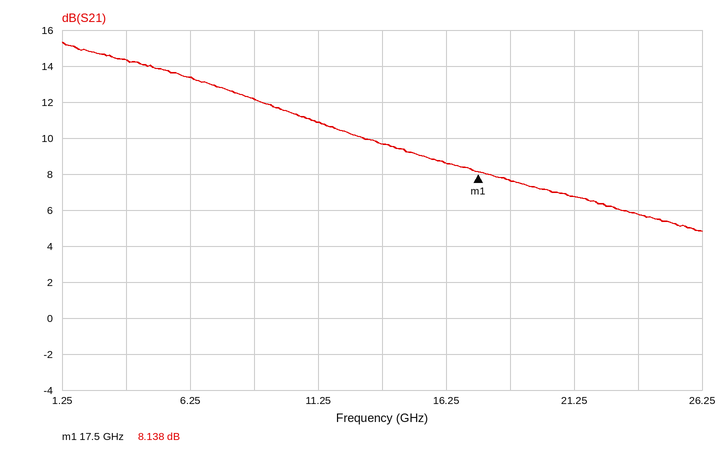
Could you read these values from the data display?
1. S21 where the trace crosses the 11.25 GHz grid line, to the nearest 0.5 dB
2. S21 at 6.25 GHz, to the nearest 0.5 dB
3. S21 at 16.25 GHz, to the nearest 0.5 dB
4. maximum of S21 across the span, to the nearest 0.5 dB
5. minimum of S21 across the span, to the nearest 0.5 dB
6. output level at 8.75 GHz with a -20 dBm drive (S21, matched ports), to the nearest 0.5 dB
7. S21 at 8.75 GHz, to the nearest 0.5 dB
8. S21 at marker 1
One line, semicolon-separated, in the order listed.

11.0 dB; 13.5 dB; 8.5 dB; 15.5 dB; 5.0 dB; -8.0 dBm; 12.0 dB; 8.138 dB
